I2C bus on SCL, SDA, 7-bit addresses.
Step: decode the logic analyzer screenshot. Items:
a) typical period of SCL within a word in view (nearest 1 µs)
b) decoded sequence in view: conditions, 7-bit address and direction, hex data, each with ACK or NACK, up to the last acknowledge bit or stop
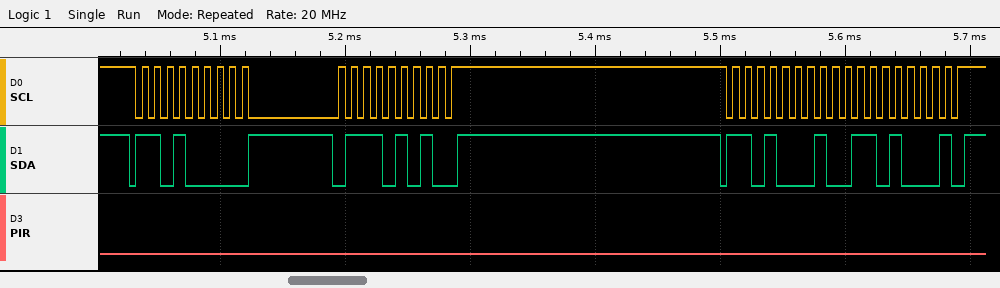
10 µs
start, address 68 write ACK, 75 ACK, stop, start, address 68 read ACK, 68 NACK, stop
